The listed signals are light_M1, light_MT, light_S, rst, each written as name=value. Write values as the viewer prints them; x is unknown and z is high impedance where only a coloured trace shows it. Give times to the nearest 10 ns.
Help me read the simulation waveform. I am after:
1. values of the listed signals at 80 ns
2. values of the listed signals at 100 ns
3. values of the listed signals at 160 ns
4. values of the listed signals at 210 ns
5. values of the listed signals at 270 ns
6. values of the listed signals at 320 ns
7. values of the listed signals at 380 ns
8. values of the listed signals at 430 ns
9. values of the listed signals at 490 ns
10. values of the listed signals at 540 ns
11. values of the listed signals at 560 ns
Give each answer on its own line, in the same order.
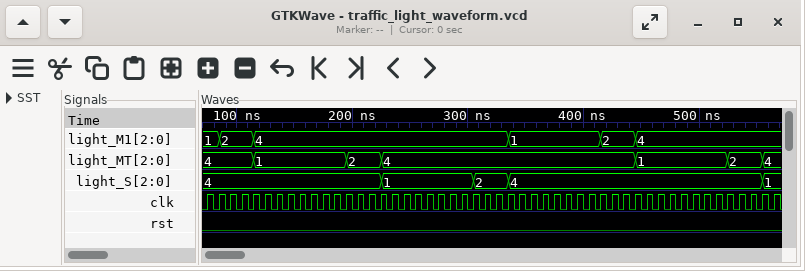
light_M1=1, light_MT=4, light_S=4, rst=0
light_M1=2, light_MT=4, light_S=4, rst=0
light_M1=4, light_MT=1, light_S=4, rst=0
light_M1=4, light_MT=2, light_S=4, rst=0
light_M1=4, light_MT=4, light_S=1, rst=0
light_M1=4, light_MT=4, light_S=2, rst=0
light_M1=1, light_MT=4, light_S=4, rst=0
light_M1=2, light_MT=4, light_S=4, rst=0
light_M1=4, light_MT=1, light_S=4, rst=0
light_M1=4, light_MT=2, light_S=4, rst=0
light_M1=4, light_MT=4, light_S=1, rst=0
